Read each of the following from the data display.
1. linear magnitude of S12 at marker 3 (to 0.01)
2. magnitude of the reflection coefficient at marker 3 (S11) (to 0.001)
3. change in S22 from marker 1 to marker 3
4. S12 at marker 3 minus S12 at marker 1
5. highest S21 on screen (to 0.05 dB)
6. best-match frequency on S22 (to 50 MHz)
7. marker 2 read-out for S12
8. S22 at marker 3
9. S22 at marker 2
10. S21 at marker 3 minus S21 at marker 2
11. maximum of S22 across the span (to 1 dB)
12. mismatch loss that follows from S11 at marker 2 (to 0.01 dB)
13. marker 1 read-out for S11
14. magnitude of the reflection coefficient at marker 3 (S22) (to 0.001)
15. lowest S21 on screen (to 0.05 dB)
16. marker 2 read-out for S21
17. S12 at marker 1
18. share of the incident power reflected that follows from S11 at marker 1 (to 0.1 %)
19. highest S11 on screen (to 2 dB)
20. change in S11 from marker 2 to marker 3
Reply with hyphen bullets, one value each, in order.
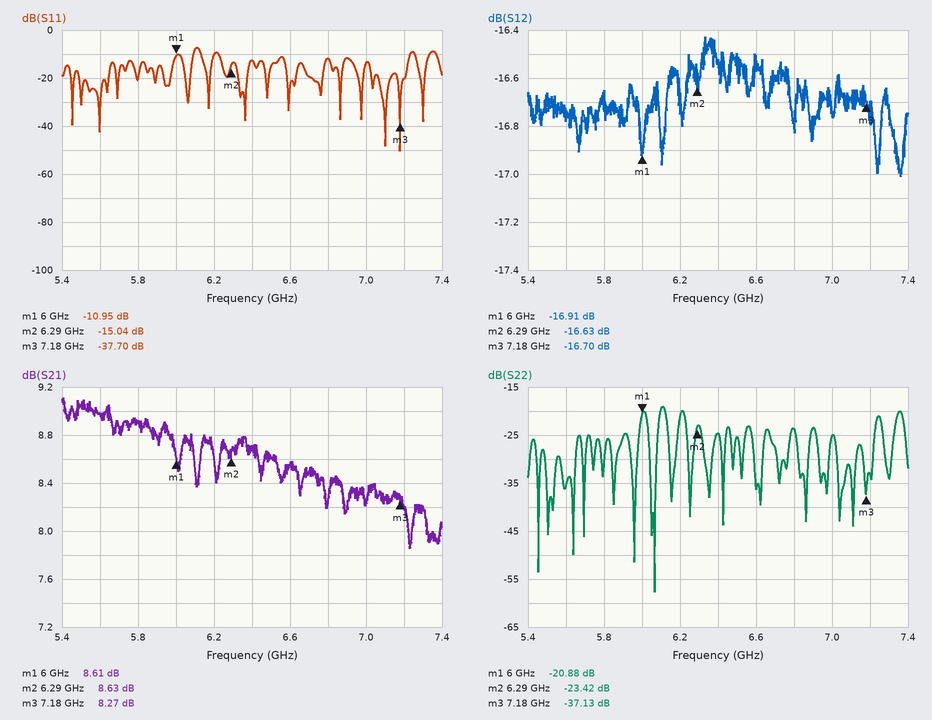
- 0.15
- 0.013
- -16.25 dB
- 0.21 dB
- 9.10 dB
- 6.05 GHz
- -16.63 dB
- -37.13 dB
- -23.42 dB
- -0.36 dB
- -19 dB
- 0.14 dB
- -10.95 dB
- 0.014
- 7.85 dB
- 8.63 dB
- -16.91 dB
- 8.0 %
- -8 dB
- -22.66 dB
